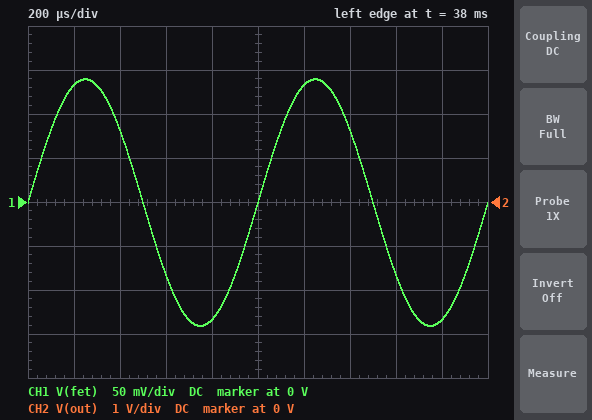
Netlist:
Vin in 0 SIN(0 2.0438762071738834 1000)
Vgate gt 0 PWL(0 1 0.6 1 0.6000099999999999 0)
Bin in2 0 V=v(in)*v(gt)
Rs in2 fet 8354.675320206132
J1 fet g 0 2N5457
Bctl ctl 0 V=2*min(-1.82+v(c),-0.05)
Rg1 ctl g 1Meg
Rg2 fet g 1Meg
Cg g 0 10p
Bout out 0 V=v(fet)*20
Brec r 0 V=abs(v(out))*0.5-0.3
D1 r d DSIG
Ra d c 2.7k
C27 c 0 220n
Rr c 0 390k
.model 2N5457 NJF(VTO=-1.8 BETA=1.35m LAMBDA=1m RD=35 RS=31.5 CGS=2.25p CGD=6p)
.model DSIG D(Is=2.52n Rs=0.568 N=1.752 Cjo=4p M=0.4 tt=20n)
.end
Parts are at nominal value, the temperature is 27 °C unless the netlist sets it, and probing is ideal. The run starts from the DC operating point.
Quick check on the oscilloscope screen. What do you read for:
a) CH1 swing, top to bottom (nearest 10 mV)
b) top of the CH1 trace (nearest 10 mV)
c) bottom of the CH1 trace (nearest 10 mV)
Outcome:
280 mV
140 mV
-140 mV
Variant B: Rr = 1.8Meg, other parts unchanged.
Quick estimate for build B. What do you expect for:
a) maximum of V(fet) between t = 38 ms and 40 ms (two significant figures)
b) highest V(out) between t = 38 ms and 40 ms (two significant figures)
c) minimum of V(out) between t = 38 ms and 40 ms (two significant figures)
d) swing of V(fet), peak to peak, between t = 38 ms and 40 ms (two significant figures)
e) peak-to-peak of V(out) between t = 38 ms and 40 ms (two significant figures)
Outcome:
130 mV
2.7 V
-2.7 V
270 mV
5.4 V
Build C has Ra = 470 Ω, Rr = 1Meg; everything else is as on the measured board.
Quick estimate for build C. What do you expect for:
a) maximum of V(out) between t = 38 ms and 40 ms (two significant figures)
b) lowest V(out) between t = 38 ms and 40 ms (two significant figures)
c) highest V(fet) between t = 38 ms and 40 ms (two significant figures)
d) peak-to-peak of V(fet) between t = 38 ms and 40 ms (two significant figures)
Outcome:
2.7 V
-2.7 V
140 mV
270 mV
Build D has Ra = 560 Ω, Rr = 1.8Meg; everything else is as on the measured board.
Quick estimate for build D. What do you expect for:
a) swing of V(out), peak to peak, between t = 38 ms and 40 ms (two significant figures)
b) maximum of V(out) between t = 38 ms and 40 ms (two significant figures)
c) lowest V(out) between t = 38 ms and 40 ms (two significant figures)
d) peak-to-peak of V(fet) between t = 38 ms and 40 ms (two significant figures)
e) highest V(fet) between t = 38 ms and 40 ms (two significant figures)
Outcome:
5.4 V
2.7 V
-2.7 V
270 mV
130 mV
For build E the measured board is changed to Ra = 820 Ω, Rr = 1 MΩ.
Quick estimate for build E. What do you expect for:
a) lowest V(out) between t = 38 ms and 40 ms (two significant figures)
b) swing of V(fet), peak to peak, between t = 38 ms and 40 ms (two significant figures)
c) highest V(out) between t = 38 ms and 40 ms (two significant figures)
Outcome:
-2.7 V
270 mV
2.7 V
